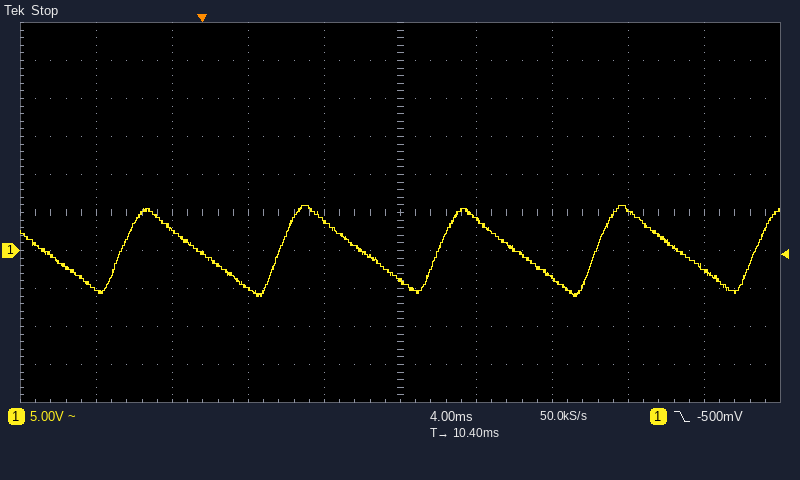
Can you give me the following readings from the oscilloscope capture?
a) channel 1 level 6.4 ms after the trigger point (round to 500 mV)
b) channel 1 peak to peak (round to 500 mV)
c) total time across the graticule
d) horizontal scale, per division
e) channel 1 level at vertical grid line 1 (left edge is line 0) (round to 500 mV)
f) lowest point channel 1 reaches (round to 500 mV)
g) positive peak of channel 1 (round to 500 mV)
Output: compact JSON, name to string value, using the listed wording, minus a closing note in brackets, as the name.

{"channel 1 level 6.4 ms after the trigger point": "4.0 V", "channel 1 peak to peak": "12.0 V", "total time across the graticule": "40 ms", "horizontal scale, per division": "4 ms", "channel 1 level at vertical grid line 1 (left edge is line 0)": "-5.5 V", "lowest point channel 1 reaches": "-6.0 V", "positive peak of channel 1": "6.0 V"}
